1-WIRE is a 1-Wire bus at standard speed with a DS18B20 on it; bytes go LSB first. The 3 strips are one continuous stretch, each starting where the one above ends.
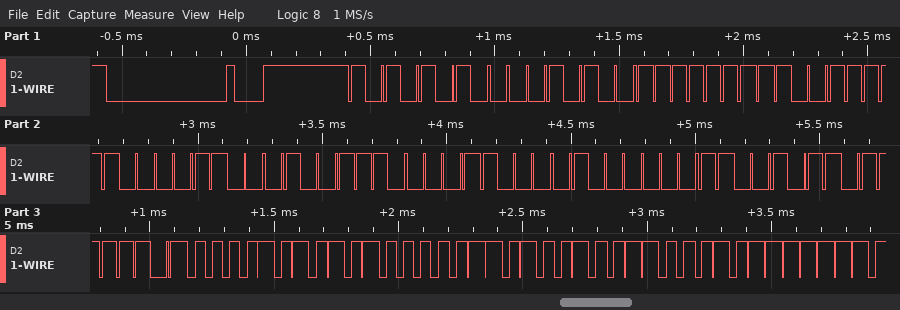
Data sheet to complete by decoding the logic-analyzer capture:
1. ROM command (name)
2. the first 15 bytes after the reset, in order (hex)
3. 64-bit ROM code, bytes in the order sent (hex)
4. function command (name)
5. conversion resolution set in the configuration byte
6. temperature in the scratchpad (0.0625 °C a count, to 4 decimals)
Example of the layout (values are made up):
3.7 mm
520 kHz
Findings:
Match ROM
55 28 FF F9 30 72 18 02 D3 BE 50 05 4B 46 7F
28 FF F9 30 72 18 02 D3
Read Scratchpad
12 bits
85.0000 °C
